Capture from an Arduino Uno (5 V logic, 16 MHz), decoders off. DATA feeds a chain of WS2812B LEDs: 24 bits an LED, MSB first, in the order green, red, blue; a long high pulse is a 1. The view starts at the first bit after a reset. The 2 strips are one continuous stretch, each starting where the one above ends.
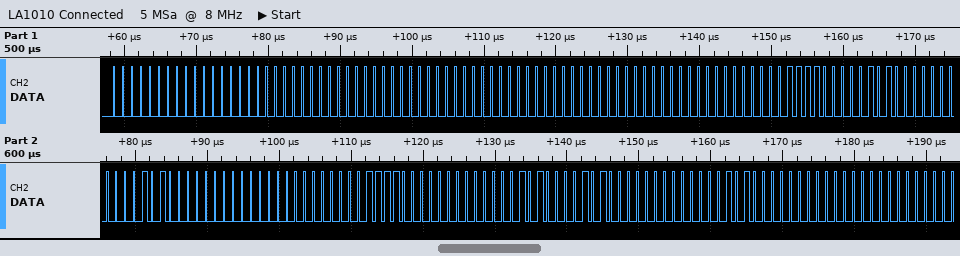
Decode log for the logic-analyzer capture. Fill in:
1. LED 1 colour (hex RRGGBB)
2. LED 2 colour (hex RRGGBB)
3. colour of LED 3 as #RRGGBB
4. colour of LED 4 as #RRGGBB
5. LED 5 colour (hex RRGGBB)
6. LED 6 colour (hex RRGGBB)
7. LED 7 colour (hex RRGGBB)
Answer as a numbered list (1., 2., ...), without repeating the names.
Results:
1. #000000
2. #000000
3. #000000
4. #0A1E00
5. #002800
6. #001E0A
7. #001414
